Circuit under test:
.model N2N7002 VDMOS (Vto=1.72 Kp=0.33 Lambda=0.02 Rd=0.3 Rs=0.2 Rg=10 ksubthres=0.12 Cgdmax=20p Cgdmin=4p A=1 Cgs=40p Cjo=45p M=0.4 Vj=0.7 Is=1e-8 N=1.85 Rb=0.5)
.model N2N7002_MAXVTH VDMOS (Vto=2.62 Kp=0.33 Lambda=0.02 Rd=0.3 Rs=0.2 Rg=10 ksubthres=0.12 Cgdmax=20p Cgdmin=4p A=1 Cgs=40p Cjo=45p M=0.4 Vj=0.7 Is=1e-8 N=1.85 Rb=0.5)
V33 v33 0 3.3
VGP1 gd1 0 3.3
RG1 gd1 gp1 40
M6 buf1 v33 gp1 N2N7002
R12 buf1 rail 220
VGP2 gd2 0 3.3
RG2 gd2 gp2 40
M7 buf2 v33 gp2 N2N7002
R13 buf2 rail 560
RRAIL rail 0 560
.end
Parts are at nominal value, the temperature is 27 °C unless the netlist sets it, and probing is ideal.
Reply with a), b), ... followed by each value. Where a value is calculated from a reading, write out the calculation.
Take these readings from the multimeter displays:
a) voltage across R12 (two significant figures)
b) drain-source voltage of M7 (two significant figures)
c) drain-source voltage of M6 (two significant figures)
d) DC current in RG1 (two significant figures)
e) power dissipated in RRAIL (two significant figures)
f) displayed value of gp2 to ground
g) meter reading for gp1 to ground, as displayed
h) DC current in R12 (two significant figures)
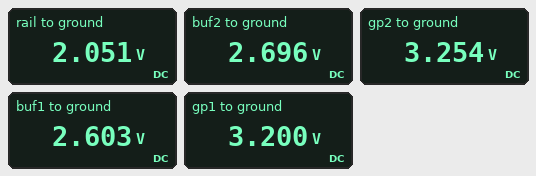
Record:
a) 2.603 V - 2.051 V = 550 mV
b) 2.696 V - 3.254 V = -560 mV
c) 2.603 V - 3.2 V = -600 mV
d) (3.3 V - 3.2 V) / 40 Ω = 2.5 mA
e) (2.051 V)^2 / 560 Ω = 7.5 mW
f) 3.254 V
g) 3.200 V
h) (2.603 V - 2.051 V) / 220 Ω = 2.5 mA
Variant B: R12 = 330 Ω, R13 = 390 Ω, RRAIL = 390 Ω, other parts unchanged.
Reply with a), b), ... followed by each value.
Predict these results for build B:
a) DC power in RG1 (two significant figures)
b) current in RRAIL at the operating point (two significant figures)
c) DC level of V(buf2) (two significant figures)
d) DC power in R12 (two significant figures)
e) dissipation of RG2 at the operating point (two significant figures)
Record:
a) 240 µW
b) 4.6 mA
c) 2.6 V
d) 2.0 mW
e) 180 µW
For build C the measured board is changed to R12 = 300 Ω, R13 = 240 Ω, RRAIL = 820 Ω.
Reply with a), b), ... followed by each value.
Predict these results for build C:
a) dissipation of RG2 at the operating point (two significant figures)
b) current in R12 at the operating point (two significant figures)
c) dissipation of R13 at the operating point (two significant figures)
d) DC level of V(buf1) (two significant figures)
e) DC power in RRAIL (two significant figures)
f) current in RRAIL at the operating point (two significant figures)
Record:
a) 93 µW
b) 1.3 mA
c) 560 µW
d) 2.7 V
e) 6.5 mW
f) 2.8 mA
